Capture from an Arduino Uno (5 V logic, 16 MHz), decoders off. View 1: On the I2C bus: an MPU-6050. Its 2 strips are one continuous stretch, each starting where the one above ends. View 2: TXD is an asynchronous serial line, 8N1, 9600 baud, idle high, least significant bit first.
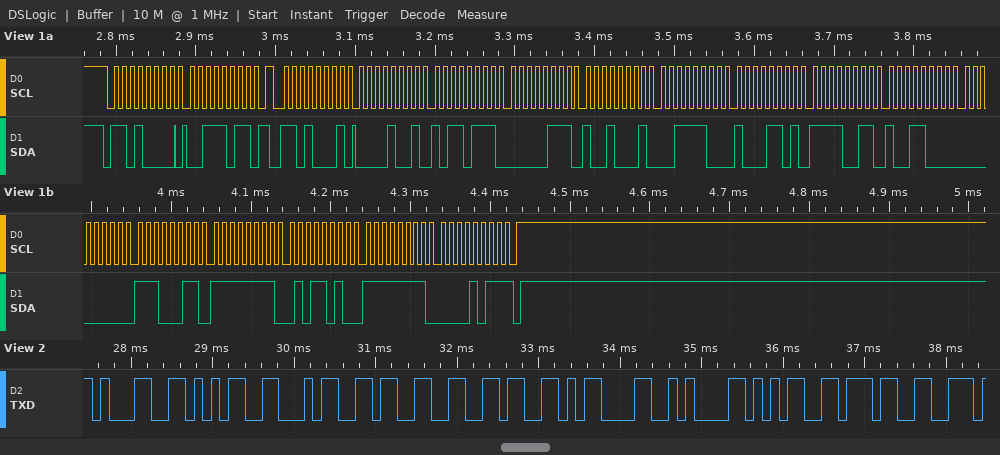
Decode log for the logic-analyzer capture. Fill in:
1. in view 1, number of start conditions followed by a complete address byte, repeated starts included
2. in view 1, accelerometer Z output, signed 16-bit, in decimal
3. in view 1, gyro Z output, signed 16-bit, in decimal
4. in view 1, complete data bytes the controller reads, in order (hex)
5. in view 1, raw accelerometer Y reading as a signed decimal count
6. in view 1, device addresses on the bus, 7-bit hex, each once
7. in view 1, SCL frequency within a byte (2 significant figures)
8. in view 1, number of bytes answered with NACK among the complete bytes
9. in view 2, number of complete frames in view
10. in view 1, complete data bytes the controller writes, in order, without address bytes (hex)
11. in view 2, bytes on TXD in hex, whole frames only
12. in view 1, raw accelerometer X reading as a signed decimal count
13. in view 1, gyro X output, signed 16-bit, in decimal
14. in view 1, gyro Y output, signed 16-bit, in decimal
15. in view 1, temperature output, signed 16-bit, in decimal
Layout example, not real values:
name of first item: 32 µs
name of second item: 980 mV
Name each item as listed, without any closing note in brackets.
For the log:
in view 1, number of start conditions followed by a complete address byte, repeated starts included: 2
in view 1, accelerometer Z output, signed 16-bit, in decimal: 15501
in view 1, gyro Z output, signed 16-bit, in decimal: -245
in view 1, complete data bytes the controller reads, in order: 09 B7 07 91 3C 8D F3 98 00 E3 FF 5A FF 0B
in view 1, raw accelerometer Y reading as a signed decimal count: 1937
in view 1, device addresses on the bus, 7-bit hex, each once: 0x68
in view 1, SCL frequency within a byte: 100 kHz
in view 1, number of bytes answered with NACK among the complete bytes: 1
in view 2, number of complete frames in view: 9
in view 1, complete data bytes the controller writes, in order, without address bytes: 3B
in view 2, bytes on TXD in hex, whole frames only: 31 35 34 33 36 0D 0A 35 37
in view 1, raw accelerometer X reading as a signed decimal count: 2487
in view 1, gyro X output, signed 16-bit, in decimal: 227
in view 1, gyro Y output, signed 16-bit, in decimal: -166
in view 1, temperature output, signed 16-bit, in decimal: -3176
